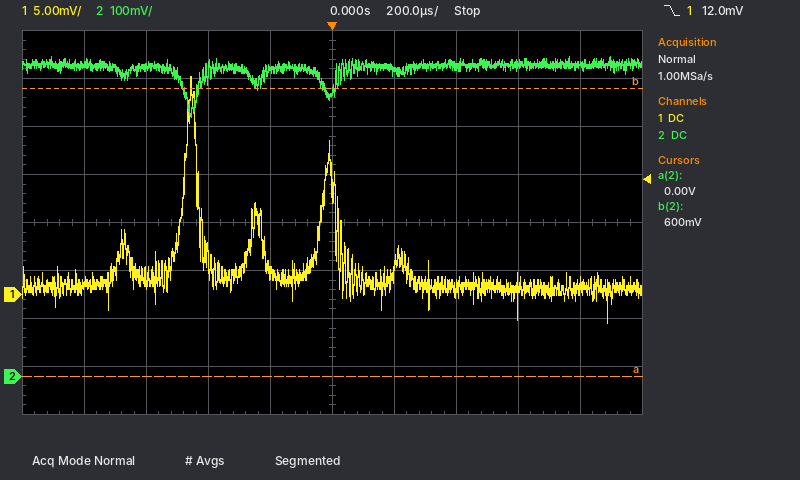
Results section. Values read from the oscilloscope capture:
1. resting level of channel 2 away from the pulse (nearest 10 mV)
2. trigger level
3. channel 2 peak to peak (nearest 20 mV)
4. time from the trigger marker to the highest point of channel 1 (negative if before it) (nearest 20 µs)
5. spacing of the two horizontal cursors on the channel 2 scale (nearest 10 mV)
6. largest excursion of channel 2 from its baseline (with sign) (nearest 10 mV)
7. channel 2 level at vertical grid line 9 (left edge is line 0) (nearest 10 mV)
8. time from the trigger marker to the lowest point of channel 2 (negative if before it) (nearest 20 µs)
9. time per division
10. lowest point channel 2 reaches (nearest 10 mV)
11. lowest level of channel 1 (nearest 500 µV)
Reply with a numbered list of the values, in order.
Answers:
1. 650 mV
2. 12.0 mV
3. 120 mV
4. -460 µs
5. 600 mV
6. -110 mV
7. 650 mV
8. -460 µs
9. 200 µs
10. 540 mV
11. -3.0 mV
